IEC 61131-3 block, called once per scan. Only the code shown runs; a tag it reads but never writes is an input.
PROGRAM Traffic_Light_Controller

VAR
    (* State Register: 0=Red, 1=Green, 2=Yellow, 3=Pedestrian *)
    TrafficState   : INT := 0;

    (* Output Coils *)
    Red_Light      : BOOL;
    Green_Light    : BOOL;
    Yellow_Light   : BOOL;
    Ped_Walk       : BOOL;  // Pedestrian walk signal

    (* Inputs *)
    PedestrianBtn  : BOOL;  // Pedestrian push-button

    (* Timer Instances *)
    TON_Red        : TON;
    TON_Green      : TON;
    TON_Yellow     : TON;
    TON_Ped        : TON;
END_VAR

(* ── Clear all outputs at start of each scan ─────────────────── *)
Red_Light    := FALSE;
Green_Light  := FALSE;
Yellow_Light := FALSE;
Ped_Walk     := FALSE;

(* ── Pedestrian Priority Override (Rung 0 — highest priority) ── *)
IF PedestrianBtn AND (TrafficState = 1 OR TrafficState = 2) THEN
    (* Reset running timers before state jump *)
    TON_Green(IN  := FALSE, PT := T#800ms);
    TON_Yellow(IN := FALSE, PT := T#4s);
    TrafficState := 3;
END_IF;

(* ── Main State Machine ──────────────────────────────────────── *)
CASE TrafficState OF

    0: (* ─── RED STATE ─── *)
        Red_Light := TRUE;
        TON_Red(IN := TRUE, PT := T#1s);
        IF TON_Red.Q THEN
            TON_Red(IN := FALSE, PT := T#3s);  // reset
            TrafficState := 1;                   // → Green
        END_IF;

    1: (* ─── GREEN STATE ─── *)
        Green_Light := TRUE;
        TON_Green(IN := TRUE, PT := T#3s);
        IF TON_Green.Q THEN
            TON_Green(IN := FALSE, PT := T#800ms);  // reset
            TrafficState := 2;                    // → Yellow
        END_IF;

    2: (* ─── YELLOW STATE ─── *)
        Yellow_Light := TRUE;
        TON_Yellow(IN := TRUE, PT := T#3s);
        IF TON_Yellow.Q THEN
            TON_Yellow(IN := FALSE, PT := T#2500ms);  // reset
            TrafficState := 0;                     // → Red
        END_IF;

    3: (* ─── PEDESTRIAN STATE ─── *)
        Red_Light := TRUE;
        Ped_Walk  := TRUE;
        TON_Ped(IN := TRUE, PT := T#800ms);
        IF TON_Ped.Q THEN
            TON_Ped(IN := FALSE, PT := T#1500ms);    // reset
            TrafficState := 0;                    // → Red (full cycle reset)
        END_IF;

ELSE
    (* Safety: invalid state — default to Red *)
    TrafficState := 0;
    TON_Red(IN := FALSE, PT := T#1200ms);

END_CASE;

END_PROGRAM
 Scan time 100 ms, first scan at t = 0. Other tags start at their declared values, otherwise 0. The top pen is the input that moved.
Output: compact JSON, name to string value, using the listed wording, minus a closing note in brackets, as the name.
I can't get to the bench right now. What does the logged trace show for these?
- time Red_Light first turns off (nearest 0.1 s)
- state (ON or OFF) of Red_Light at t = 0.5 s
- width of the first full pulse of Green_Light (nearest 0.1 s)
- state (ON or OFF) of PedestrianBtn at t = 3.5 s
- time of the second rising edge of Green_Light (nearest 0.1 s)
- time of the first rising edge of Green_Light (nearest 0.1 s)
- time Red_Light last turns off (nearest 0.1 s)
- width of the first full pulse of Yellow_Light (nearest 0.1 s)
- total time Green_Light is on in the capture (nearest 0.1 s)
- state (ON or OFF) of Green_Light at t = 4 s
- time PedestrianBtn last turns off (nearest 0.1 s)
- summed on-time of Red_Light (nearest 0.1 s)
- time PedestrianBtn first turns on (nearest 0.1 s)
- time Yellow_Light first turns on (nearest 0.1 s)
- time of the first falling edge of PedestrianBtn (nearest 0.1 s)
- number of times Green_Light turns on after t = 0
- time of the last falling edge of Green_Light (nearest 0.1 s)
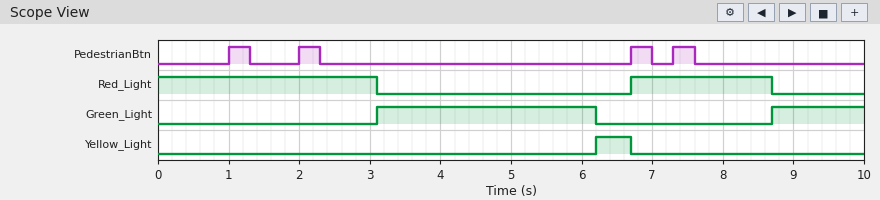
{"time Red_Light first turns off": "3.1 s", "state (ON or OFF) of Red_Light at t = 0.5 s": "ON", "width of the first full pulse of Green_Light": "3.1 s", "state (ON or OFF) of PedestrianBtn at t = 3.5 s": "OFF", "time of the second rising edge of Green_Light": "8.7 s", "time of the first rising edge of Green_Light": "3.1 s", "time Red_Light last turns off": "8.7 s", "width of the first full pulse of Yellow_Light": "0.5 s", "total time Green_Light is on in the capture": "4.4 s", "state (ON or OFF) of Green_Light at t = 4 s": "ON", "time PedestrianBtn last turns off": "7.6 s", "summed on-time of Red_Light": "5.1 s", "time PedestrianBtn first turns on": "1.0 s", "time Yellow_Light first turns on": "6.2 s", "time of the first falling edge of PedestrianBtn": "1.3 s", "number of times Green_Light turns on after t = 0": "2", "time of the last falling edge of Green_Light": "6.2 s"}
